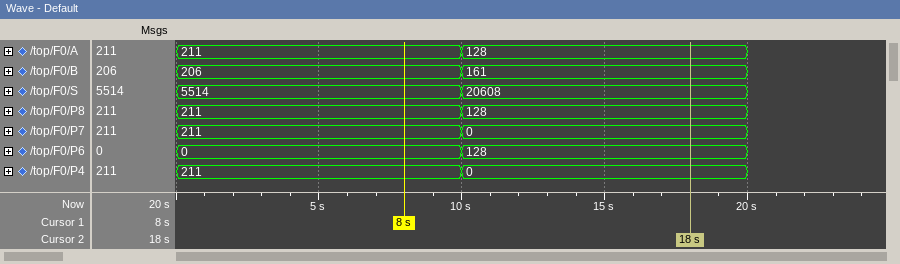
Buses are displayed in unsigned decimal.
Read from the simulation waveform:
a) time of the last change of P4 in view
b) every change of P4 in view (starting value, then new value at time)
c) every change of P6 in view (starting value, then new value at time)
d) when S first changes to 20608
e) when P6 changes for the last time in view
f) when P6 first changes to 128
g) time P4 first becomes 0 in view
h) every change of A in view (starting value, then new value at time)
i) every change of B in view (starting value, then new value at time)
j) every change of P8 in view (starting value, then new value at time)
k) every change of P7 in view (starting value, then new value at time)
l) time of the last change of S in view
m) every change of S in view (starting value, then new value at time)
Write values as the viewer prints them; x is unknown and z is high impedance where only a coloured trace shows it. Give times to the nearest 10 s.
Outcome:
10 s
211, 0 at 10 s
0, 128 at 10 s
10 s
10 s
10 s
10 s
211, 128 at 10 s
206, 161 at 10 s
211, 128 at 10 s
211, 0 at 10 s
10 s
5514, 20608 at 10 s
